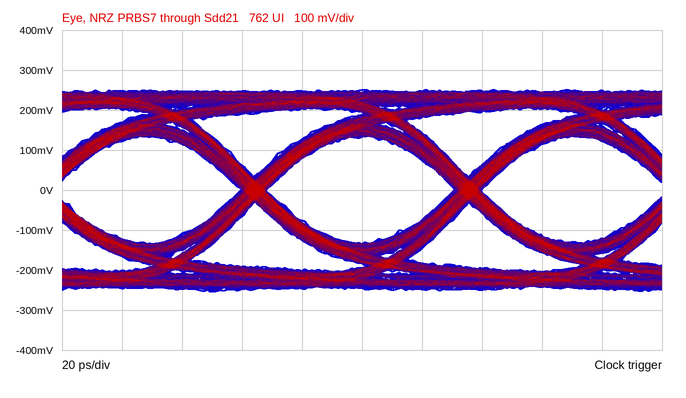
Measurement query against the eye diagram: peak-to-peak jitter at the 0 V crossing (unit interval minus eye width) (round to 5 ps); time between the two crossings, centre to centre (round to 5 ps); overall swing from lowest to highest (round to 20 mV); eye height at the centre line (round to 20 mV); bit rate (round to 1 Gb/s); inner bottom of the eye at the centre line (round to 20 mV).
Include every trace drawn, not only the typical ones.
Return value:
10 ps
70 ps
500 mV
260 mV
14 Gb/s
-140 mV
